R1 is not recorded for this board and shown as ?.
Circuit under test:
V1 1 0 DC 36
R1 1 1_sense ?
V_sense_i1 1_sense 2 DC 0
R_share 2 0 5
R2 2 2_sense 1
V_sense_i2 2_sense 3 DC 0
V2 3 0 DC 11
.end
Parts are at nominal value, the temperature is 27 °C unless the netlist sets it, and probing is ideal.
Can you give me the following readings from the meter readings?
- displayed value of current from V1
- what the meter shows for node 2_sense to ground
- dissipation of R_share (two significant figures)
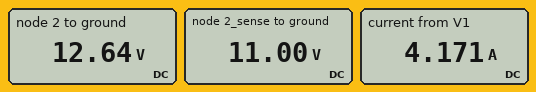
4.171 A
11.00 V
32 W
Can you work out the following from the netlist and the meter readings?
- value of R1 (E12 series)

5.6 Ω
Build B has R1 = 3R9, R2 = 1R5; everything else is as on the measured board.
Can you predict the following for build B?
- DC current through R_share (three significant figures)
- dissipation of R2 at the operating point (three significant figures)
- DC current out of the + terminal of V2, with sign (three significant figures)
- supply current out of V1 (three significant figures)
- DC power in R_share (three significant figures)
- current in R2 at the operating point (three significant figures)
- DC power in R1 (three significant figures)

2.95 A
9.37 W
-2.50 A
5.45 A
43.5 W
2.50 A
116 W
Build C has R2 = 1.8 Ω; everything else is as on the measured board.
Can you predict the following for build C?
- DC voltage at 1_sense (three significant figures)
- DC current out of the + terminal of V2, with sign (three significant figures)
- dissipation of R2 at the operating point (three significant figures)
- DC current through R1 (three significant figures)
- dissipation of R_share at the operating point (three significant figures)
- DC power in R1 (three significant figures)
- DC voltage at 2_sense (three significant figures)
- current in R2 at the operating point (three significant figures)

13.4 V
-1.35 A
3.26 W
4.03 A
36.0 W
91.0 W
11.0 V
1.35 A
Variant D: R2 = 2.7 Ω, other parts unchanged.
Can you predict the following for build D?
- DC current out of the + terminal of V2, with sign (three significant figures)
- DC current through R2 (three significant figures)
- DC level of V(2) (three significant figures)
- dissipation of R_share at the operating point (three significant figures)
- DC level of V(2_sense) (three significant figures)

-1.12 A
1.12 A
14.0 V
39.3 W
11.0 V
